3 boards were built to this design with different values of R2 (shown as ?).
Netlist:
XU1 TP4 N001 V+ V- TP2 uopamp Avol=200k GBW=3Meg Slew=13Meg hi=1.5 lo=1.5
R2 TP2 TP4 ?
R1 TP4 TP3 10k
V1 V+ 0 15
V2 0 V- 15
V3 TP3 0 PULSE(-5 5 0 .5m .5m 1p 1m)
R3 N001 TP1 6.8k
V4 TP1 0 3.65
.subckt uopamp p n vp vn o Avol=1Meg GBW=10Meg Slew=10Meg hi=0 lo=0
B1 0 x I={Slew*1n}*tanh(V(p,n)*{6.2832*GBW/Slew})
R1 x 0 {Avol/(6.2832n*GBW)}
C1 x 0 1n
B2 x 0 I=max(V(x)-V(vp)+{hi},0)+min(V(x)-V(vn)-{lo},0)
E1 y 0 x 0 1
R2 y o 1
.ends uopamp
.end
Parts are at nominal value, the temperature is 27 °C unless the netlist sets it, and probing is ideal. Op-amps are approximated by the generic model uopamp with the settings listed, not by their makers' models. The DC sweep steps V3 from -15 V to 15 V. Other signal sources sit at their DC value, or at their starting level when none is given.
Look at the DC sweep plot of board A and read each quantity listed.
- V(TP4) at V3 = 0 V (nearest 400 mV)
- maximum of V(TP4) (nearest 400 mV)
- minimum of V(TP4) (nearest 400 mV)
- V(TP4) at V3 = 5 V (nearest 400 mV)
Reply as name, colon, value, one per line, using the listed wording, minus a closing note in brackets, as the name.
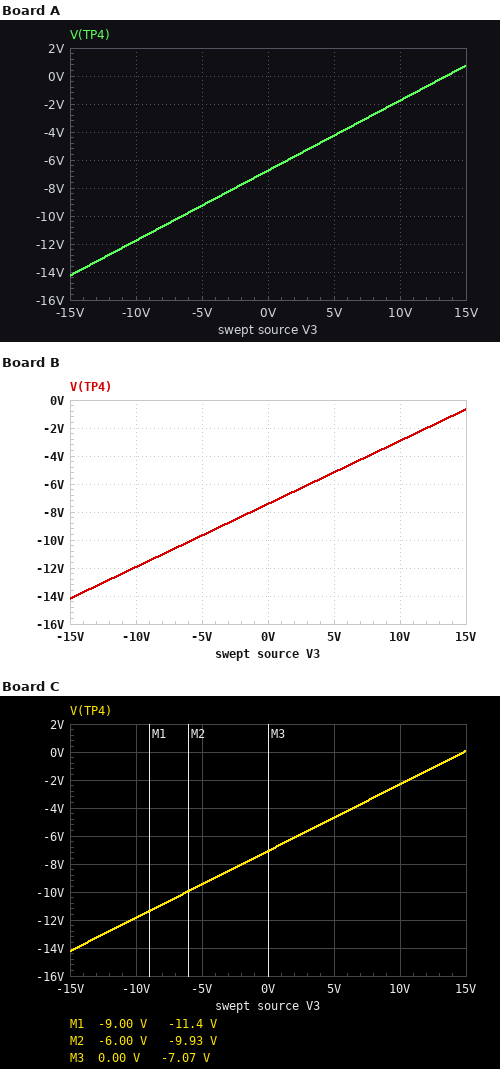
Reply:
V(TP4) at V3 = 0 V: -6.8 V
maximum of V(TP4): 800 mV
minimum of V(TP4): -14.4 V
V(TP4) at V3 = 5 V: -4.4 V
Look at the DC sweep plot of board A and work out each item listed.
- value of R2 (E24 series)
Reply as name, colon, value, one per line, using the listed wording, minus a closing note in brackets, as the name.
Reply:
value of R2: 10 kΩ
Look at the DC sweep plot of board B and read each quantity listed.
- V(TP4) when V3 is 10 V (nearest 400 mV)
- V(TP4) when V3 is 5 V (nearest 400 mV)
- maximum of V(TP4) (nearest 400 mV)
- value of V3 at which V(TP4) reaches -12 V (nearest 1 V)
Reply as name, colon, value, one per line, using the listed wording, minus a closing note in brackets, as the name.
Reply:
V(TP4) when V3 is 10 V: -2.8 V
V(TP4) when V3 is 5 V: -5.2 V
maximum of V(TP4): -800 mV
value of V3 at which V(TP4) reaches -12 V: -10 V
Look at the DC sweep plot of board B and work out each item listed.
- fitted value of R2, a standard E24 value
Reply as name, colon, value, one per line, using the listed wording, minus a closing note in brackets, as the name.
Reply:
fitted value of R2, a standard E24 value: 8.2 kΩ
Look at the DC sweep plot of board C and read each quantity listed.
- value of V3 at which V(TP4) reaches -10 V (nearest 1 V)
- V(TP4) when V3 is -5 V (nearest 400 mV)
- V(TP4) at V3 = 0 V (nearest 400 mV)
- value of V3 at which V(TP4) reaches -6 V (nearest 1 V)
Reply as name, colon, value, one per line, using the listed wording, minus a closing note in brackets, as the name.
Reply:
value of V3 at which V(TP4) reaches -10 V: -6 V
V(TP4) when V3 is -5 V: -9.6 V
V(TP4) at V3 = 0 V: -7.2 V
value of V3 at which V(TP4) reaches -6 V: 2 V
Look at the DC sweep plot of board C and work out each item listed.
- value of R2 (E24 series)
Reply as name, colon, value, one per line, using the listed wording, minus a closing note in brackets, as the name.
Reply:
value of R2: 9.1 kΩ
